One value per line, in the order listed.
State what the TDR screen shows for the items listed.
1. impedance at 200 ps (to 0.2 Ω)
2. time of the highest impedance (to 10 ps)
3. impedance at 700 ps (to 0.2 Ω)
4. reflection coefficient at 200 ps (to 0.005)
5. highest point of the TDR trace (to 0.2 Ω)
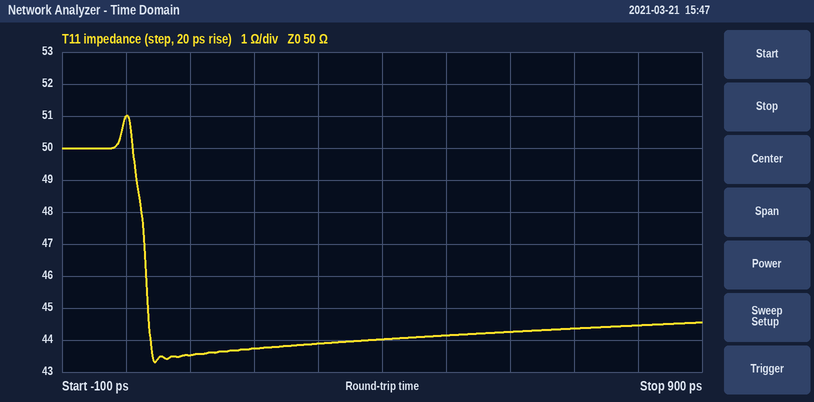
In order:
43.8 Ω
0 ps
44.4 Ω
-0.065
51.0 Ω
